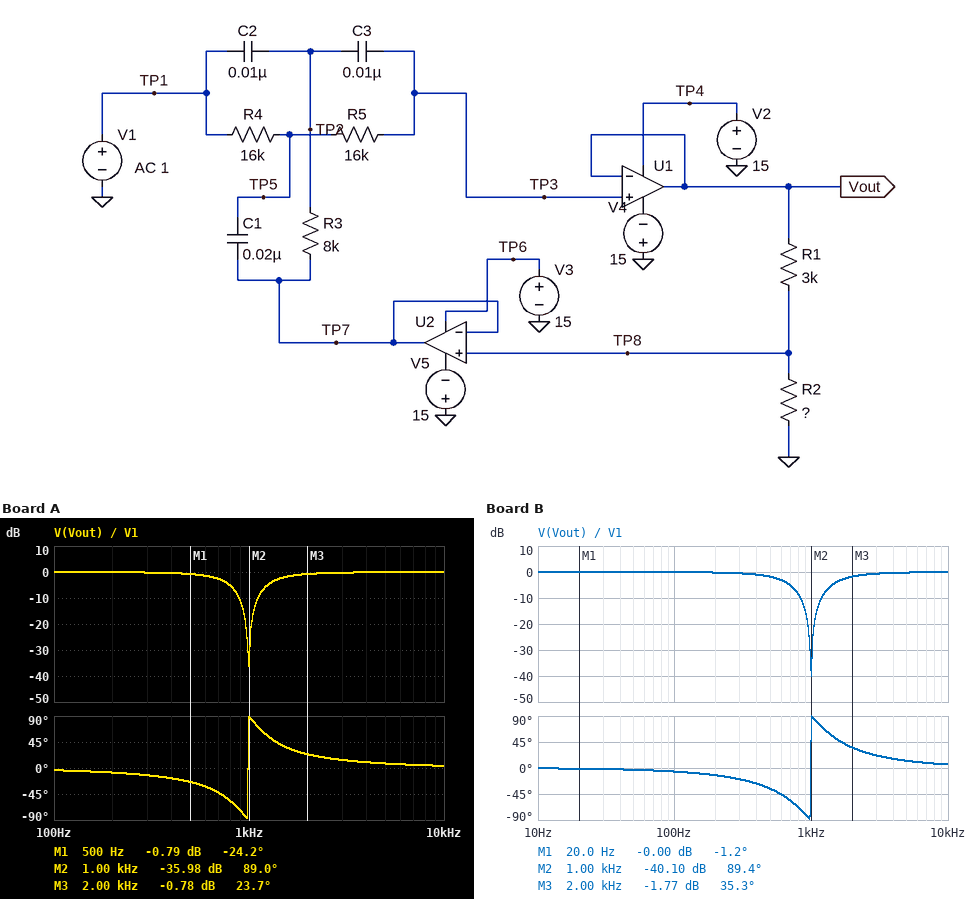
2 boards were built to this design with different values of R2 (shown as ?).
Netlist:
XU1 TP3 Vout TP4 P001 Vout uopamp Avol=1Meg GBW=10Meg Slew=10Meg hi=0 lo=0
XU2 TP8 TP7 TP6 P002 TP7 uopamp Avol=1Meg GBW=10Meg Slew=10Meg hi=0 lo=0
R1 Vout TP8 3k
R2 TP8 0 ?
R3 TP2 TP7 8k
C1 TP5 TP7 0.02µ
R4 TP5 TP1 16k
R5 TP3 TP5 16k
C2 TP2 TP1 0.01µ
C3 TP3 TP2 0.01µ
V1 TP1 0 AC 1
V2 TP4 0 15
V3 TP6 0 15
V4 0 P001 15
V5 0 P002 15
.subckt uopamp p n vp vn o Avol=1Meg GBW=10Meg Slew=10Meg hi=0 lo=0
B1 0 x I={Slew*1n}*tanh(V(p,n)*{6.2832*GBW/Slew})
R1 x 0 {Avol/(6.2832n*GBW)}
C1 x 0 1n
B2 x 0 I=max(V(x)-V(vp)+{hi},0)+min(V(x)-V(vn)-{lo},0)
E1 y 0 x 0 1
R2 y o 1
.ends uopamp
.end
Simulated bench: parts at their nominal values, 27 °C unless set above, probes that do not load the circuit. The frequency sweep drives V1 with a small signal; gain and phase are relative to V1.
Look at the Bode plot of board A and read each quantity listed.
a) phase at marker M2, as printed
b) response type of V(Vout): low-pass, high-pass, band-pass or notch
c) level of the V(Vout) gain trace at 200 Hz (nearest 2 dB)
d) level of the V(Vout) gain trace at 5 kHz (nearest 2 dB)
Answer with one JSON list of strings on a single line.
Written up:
["89.0 deg", "notch", "0 dB", "0 dB"]
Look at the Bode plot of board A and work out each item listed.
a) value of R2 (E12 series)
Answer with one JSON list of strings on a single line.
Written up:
["15 kΩ"]
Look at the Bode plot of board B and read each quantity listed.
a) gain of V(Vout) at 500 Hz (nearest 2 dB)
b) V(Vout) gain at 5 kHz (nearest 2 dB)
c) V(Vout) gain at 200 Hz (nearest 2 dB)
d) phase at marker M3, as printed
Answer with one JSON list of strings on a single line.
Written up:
["-2 dB", "0 dB", "0 dB", "35.3 deg"]
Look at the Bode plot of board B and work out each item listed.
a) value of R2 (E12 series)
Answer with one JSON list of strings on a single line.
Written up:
["8.2 kΩ"]
